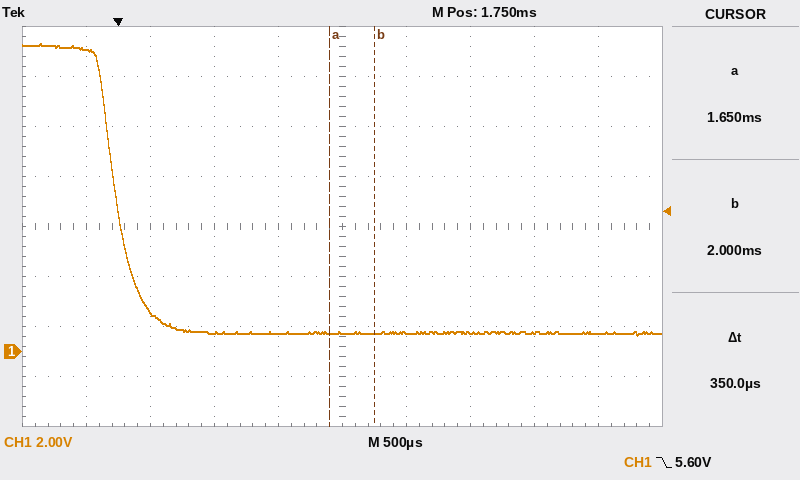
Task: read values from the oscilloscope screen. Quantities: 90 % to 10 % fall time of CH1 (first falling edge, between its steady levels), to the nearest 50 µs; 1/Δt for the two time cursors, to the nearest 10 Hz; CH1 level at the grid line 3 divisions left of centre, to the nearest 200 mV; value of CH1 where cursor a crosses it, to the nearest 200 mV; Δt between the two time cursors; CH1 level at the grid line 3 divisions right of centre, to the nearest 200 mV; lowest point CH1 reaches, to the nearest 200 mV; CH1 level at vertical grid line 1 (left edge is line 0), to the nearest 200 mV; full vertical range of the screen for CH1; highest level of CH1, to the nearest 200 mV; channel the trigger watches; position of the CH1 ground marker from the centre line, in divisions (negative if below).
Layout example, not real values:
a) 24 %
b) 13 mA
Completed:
a) 350 µs
b) 2.86 kHz
c) 1.6 V
d) 800 mV
e) 350 µs
f) 800 mV
g) 600 mV
h) 12.0 V
i) 16 V
j) 12.4 V
k) CH1
l) -2.5 div
